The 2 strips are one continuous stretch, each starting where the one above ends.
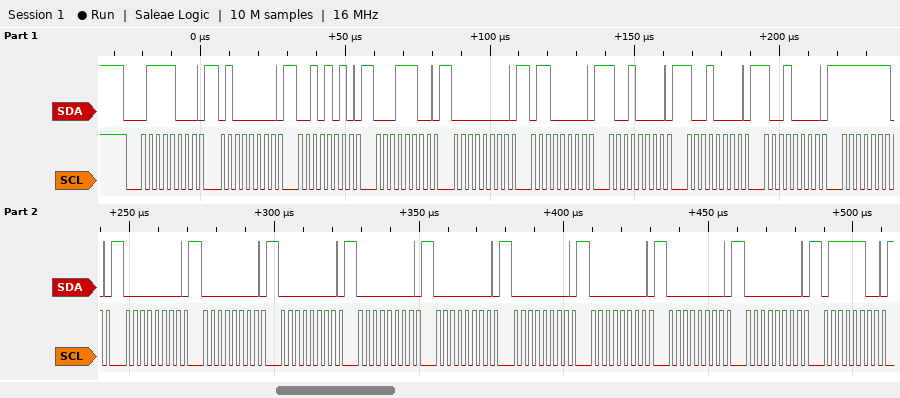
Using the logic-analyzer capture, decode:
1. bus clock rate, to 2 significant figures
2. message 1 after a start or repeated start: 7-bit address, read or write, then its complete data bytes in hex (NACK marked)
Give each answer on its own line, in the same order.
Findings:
400 kHz
0x3C write: 40 2A 1C 00 60 90 90 90 FE 00 00 00 00 00 00 00 00 00 7C
